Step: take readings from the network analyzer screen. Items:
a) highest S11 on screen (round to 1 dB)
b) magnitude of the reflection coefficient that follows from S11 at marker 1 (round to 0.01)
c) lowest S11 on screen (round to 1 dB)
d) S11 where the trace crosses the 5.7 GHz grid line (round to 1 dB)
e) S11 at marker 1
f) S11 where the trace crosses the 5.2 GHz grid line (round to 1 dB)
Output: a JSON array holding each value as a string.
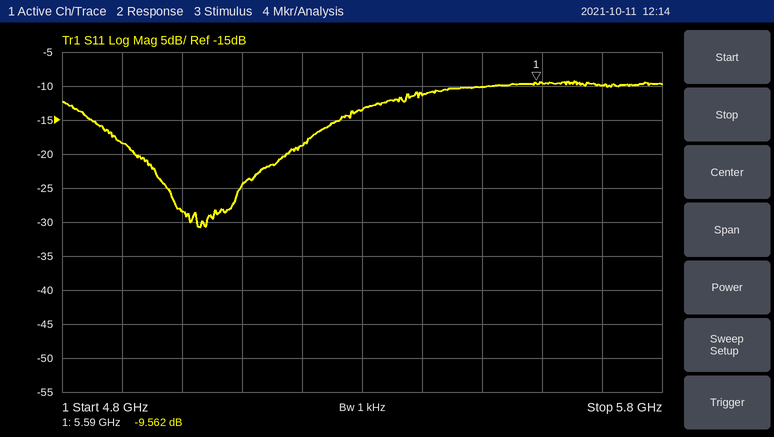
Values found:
["-9 dB", "0.33", "-31 dB", "-10 dB", "-9.562 dB", "-19 dB"]
